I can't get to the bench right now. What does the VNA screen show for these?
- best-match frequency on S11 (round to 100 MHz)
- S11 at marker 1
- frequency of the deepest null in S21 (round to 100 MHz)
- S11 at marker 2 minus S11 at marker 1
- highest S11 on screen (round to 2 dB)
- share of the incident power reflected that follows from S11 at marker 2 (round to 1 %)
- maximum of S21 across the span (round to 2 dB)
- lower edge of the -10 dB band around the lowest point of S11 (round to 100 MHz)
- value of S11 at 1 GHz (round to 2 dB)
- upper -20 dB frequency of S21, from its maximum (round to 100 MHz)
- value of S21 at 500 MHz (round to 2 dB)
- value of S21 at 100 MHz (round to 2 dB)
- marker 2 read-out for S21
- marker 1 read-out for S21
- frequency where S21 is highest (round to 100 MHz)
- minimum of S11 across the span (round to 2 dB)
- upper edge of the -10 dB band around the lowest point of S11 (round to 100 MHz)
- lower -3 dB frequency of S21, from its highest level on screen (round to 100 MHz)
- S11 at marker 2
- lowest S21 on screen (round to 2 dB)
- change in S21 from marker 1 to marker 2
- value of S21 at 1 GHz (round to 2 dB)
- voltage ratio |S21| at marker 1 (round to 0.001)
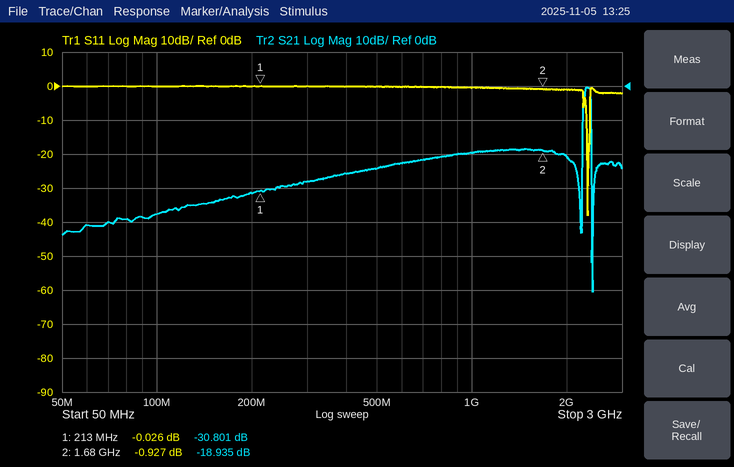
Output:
2.3 GHz
-0.026 dB
2.4 GHz
-0.901 dB
0 dB
81 %
0 dB
2.3 GHz
0 dB
2.4 GHz
-24 dB
-38 dB
-18.935 dB
-30.801 dB
2.3 GHz
-38 dB
2.4 GHz
2.3 GHz
-0.927 dB
-60 dB
11.866 dB
-20 dB
0.029
